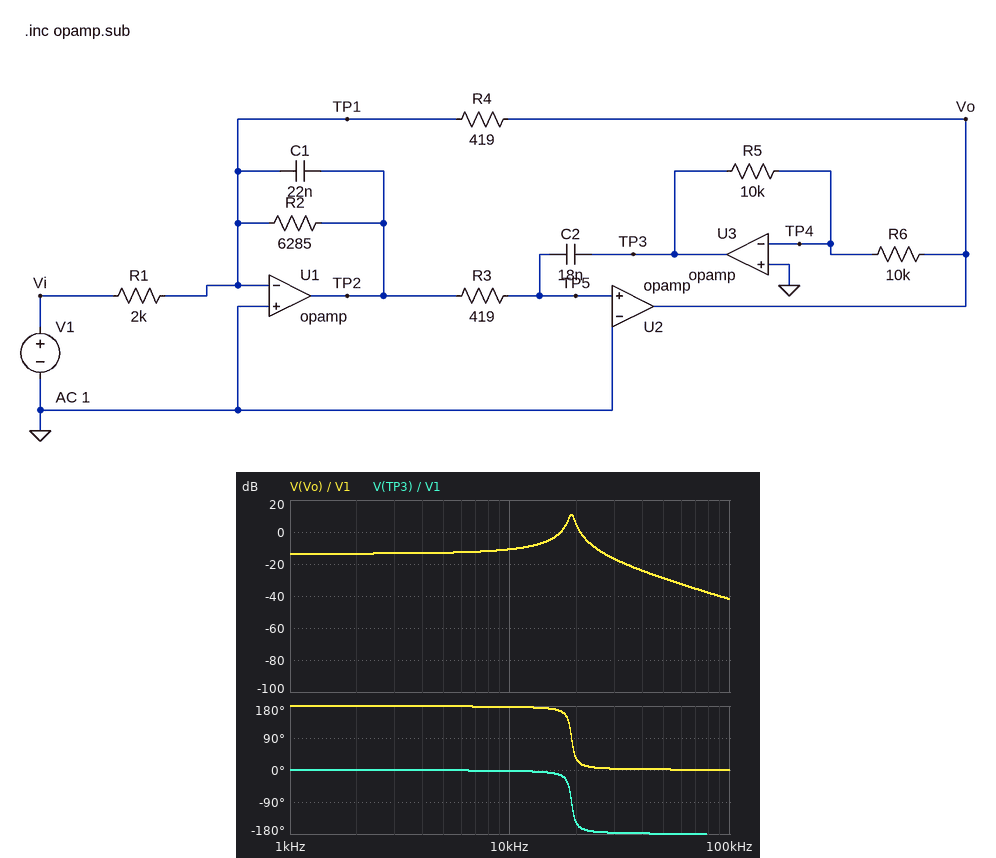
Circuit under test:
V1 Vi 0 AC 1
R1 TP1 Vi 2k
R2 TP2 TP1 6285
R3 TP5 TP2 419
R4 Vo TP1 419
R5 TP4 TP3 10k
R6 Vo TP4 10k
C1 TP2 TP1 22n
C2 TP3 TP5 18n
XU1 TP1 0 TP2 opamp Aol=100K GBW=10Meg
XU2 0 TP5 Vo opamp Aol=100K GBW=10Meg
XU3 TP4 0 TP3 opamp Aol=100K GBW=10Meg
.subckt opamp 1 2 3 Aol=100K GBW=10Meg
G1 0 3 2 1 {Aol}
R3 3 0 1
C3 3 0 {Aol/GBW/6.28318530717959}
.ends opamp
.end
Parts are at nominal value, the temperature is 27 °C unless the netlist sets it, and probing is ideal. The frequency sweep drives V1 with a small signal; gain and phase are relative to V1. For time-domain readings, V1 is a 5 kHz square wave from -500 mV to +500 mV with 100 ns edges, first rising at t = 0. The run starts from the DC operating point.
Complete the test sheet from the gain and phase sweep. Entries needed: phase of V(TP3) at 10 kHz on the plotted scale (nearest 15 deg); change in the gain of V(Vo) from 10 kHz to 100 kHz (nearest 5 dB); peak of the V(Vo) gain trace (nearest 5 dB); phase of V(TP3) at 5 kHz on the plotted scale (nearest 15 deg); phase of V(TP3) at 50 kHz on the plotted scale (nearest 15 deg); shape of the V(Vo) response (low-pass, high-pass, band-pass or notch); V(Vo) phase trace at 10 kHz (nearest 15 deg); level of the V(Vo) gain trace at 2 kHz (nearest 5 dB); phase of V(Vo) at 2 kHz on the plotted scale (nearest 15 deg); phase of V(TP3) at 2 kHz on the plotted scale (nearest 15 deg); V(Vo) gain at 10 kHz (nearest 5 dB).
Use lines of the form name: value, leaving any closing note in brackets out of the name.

phase of V(TP3) at 10 kHz on the plotted scale: 0 deg
change in the gain of V(Vo) from 10 kHz to 100 kHz: -30 dB
peak of the V(Vo) gain trace: 10 dB
phase of V(TP3) at 5 kHz on the plotted scale: 0 deg
phase of V(TP3) at 50 kHz on the plotted scale: -180 deg
shape of the V(Vo) response: low-pass
V(Vo) phase trace at 10 kHz: 180 deg
level of the V(Vo) gain trace at 2 kHz: -15 dB
phase of V(Vo) at 2 kHz on the plotted scale: 180 deg
phase of V(TP3) at 2 kHz on the plotted scale: 0 deg
V(Vo) gain at 10 kHz: -10 dB
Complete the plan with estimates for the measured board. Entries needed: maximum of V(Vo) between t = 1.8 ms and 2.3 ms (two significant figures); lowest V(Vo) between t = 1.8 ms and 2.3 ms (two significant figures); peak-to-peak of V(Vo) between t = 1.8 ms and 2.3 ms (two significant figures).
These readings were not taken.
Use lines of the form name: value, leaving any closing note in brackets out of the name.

maximum of V(Vo) between t = 1.8 ms and 2.3 ms: 220 mV
lowest V(Vo) between t = 1.8 ms and 2.3 ms: -220 mV
peak-to-peak of V(Vo) between t = 1.8 ms and 2.3 ms: 450 mV
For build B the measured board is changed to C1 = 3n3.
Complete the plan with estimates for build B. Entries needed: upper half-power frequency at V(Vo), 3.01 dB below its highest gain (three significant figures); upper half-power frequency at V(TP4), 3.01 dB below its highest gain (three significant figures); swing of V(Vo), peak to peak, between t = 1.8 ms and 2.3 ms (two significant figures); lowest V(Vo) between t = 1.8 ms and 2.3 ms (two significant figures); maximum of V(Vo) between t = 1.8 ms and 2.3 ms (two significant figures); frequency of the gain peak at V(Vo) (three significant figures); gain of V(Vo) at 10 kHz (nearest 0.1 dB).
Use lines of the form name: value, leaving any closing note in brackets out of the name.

upper half-power frequency at V(Vo), 3.01 dB below its highest gain: 52.3 kHz
upper half-power frequency at V(TP4), 3.01 dB below its highest gain: 52.8 kHz
swing of V(Vo), peak to peak, between t = 1.8 ms and 2.3 ms: 520 mV
lowest V(Vo) between t = 1.8 ms and 2.3 ms: -260 mV
maximum of V(Vo) between t = 1.8 ms and 2.3 ms: 260 mV
frequency of the gain peak at V(Vo): 48.6 kHz
gain of V(Vo) at 10 kHz: -13.2 dB
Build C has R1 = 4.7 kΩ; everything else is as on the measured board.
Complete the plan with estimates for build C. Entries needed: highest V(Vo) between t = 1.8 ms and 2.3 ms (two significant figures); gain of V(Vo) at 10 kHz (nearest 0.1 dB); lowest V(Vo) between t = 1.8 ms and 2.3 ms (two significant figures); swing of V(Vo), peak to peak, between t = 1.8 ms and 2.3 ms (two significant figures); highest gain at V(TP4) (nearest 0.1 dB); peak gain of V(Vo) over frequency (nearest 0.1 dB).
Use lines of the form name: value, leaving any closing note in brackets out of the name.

highest V(Vo) between t = 1.8 ms and 2.3 ms: 95 mV
gain of V(Vo) at 10 kHz: -18.2 dB
lowest V(Vo) between t = 1.8 ms and 2.3 ms: -95 mV
swing of V(Vo), peak to peak, between t = 1.8 ms and 2.3 ms: 190 mV
highest gain at V(TP4): -51.0 dB
peak gain of V(Vo) over frequency: 3.4 dB
